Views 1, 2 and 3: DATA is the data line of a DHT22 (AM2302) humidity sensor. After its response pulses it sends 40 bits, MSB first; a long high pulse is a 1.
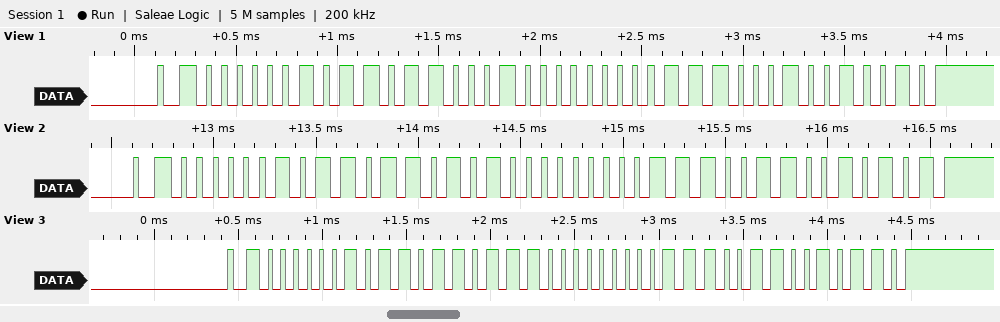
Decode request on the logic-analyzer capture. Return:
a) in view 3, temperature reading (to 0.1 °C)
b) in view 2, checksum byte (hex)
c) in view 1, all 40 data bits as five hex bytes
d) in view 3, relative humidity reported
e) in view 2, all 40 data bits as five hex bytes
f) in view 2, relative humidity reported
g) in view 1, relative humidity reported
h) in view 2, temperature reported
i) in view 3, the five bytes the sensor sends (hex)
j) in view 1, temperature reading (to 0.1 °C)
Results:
-5.7 °C
0x95
02 D8 80 38 92
73.1 %
02 DA 80 39 95
73.0 %
72.8 %
-5.7 °C
02 DB 80 39 96
-5.6 °C
